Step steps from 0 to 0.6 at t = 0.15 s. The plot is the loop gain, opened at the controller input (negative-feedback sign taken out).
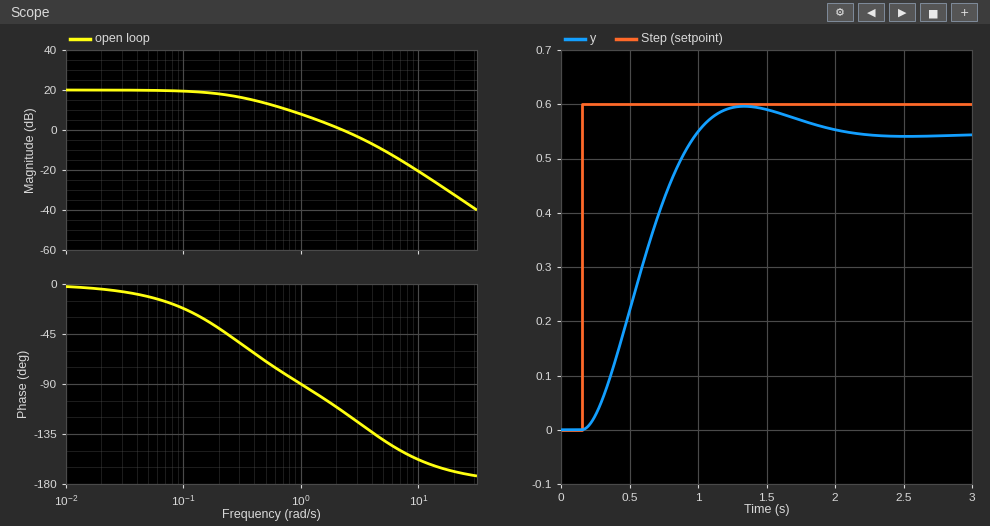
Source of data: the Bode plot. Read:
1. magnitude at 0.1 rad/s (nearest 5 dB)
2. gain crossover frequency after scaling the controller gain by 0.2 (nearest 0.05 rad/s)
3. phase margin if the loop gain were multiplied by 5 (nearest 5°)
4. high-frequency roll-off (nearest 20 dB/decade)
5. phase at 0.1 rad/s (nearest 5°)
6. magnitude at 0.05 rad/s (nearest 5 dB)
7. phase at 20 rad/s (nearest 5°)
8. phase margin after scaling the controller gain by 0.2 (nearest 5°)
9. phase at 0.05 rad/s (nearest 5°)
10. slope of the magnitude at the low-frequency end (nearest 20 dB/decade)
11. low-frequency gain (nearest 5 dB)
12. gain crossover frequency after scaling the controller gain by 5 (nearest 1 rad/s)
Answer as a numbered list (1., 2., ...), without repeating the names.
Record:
1. 20 dB
2. 0.45 rad/s
3. 30°
4. -40 dB/decade
5. -20°
6. 20 dB
7. -170°
8. 115°
9. -10°
10. 0 dB/decade
11. 20 dB
12. 7 rad/s
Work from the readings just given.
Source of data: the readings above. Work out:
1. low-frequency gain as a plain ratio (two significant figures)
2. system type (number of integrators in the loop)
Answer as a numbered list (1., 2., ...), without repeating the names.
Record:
1. 10
2. 0
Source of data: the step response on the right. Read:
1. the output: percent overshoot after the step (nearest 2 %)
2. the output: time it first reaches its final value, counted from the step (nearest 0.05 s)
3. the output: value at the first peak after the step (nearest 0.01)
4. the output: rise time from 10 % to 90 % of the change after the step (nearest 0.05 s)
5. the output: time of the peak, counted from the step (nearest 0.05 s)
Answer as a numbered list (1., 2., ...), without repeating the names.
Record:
1. 10 %
2. 0.85 s
3. 0.60
4. 0.55 s
5. 1.20 s
